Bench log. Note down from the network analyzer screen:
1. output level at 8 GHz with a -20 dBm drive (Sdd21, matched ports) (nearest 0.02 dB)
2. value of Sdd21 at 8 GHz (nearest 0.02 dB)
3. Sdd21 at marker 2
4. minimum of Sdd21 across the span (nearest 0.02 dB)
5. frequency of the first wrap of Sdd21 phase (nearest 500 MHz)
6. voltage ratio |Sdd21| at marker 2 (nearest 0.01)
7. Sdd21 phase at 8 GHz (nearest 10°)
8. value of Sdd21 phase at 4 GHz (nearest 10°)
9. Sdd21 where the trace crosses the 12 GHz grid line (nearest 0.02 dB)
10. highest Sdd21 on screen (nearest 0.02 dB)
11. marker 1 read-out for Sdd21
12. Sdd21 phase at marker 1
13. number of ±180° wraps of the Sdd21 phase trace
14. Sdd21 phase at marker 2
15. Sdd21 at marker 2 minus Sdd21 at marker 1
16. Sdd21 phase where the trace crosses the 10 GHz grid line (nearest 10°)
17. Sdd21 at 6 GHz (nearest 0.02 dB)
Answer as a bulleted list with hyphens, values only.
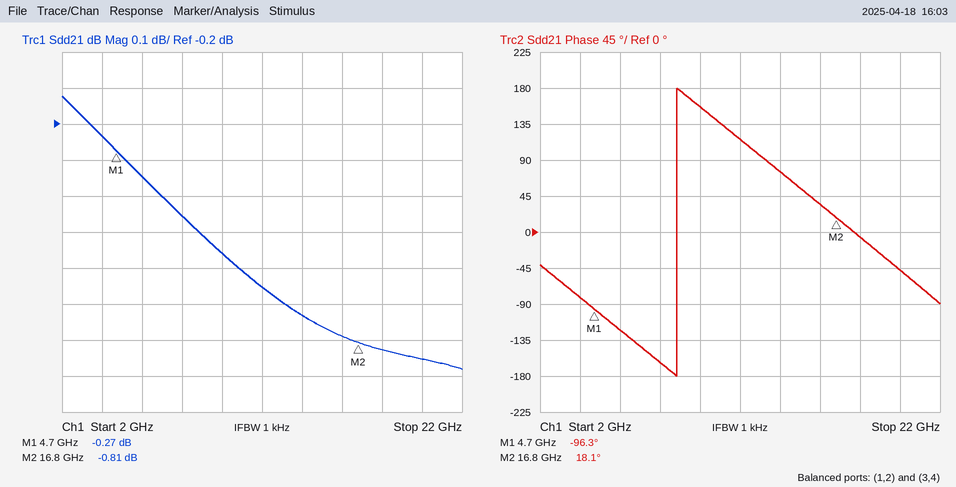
- -20.46 dBm
- -0.46 dB
- -0.81 dB
- -0.88 dB
- 9.0 GHz
- 0.91
- -160°
- -80°
- -0.66 dB
- -0.12 dB
- -0.27 dB
- -96.3°
- 1
- 18.1°
- -0.54 dB
- 160°
- -0.34 dB
